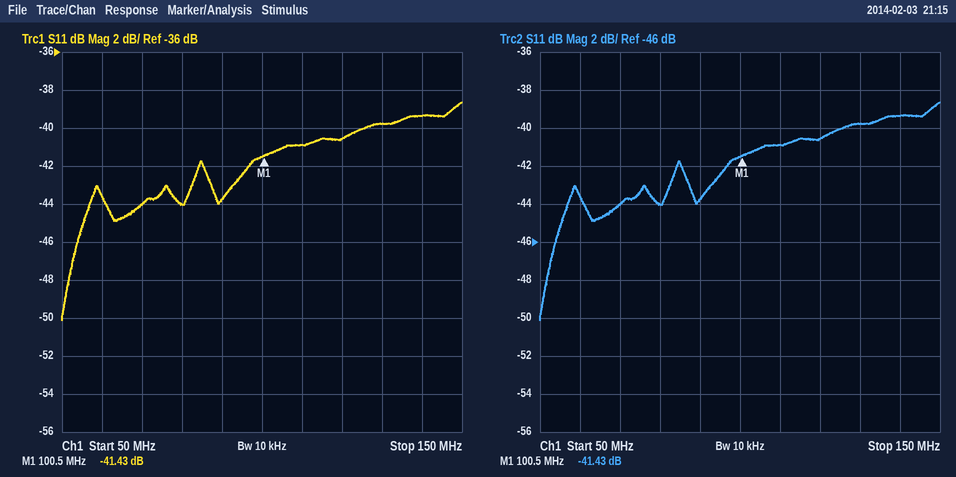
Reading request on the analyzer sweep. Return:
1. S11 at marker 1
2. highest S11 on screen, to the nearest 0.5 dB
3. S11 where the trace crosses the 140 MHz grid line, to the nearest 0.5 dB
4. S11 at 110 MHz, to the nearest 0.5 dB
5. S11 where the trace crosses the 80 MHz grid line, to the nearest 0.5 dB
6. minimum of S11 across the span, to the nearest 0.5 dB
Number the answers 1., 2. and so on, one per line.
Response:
1. -41.43 dB
2. -38.5 dB
3. -39.5 dB
4. -41.0 dB
5. -44.0 dB
6. -50.0 dB
